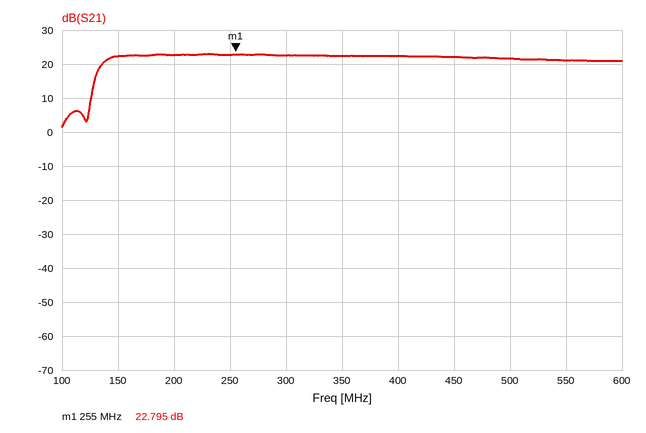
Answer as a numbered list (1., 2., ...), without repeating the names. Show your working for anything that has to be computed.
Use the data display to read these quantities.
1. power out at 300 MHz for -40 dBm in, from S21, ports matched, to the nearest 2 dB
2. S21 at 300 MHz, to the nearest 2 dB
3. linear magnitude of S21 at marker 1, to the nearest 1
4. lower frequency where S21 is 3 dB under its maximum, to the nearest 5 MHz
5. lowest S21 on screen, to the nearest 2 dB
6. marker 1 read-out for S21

1. -40 dBm + (22 dB) = -18 dBm
2. 22 dB
3. 10^(22.795/20) ≈ 14
4. 135 MHz
5. 2 dB
6. 22.795 dB
